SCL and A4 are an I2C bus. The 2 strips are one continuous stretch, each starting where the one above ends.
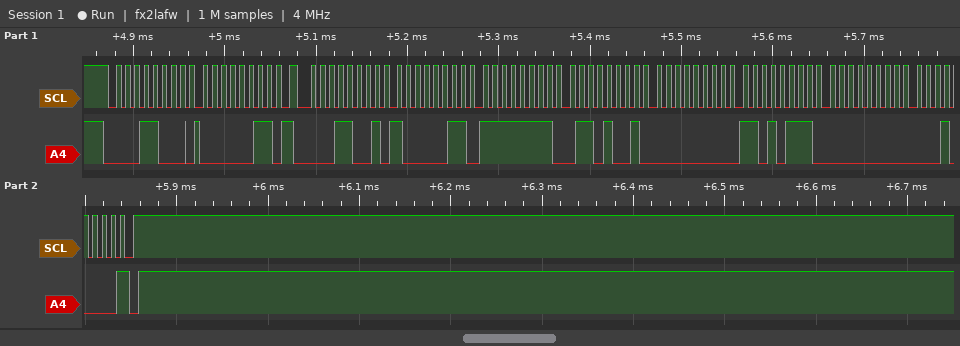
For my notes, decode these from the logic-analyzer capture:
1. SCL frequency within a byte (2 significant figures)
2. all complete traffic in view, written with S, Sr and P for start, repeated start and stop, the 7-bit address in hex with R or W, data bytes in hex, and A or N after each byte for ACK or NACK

100 kHz
S 0CW A 03 A Sr 0CR A 83 A FF A 69 A 00 A D7 A 00 A 10 N P
